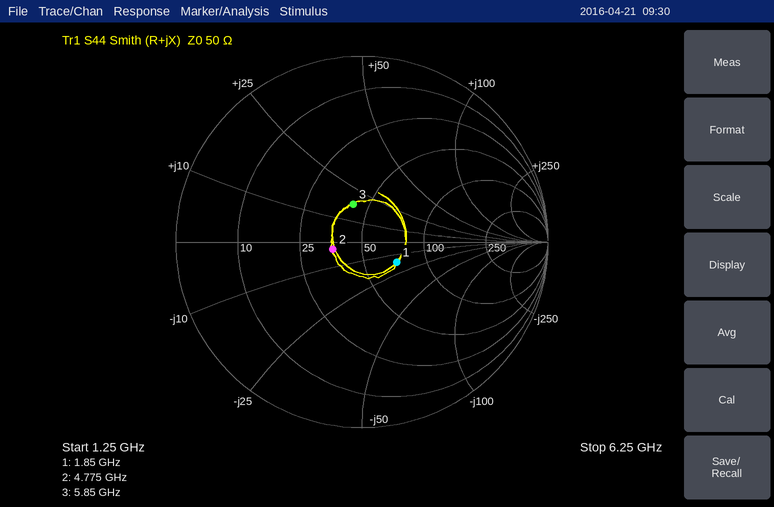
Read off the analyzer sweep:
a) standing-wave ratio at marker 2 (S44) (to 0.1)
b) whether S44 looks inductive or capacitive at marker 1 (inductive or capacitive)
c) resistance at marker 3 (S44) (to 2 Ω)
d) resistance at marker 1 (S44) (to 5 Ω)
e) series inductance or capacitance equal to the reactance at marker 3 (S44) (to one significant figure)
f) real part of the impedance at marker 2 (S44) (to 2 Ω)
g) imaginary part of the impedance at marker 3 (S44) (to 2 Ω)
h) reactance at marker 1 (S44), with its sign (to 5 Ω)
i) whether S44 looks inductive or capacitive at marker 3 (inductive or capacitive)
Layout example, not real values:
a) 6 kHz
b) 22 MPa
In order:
a) 1.4
b) capacitive
c) 42 Ω
d) 70 Ω
e) 500 pH
f) 36 Ω
g) +18 Ω
h) -15 Ω
i) inductive
